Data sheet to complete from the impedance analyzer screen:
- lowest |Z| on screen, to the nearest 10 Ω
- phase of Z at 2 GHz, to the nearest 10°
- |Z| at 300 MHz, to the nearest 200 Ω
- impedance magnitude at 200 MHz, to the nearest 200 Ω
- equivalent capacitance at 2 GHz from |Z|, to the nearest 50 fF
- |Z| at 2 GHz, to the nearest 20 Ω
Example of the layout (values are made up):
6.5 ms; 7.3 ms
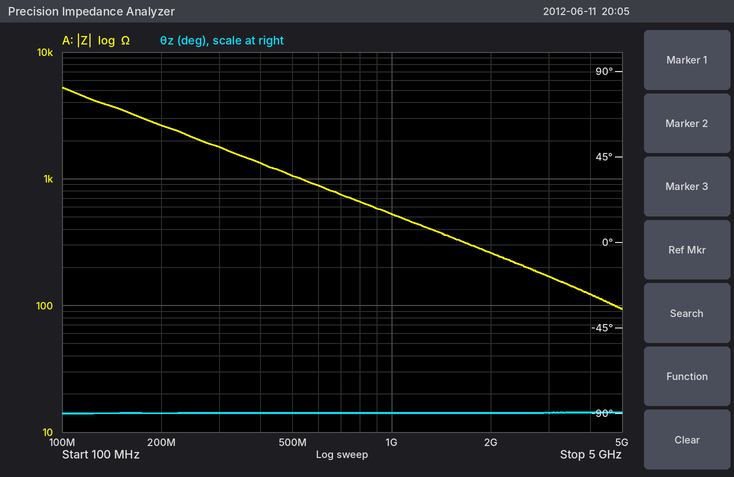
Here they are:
90 Ω; -90°; 1.8 kΩ; 2.6 kΩ; 300 fF; 260 Ω
